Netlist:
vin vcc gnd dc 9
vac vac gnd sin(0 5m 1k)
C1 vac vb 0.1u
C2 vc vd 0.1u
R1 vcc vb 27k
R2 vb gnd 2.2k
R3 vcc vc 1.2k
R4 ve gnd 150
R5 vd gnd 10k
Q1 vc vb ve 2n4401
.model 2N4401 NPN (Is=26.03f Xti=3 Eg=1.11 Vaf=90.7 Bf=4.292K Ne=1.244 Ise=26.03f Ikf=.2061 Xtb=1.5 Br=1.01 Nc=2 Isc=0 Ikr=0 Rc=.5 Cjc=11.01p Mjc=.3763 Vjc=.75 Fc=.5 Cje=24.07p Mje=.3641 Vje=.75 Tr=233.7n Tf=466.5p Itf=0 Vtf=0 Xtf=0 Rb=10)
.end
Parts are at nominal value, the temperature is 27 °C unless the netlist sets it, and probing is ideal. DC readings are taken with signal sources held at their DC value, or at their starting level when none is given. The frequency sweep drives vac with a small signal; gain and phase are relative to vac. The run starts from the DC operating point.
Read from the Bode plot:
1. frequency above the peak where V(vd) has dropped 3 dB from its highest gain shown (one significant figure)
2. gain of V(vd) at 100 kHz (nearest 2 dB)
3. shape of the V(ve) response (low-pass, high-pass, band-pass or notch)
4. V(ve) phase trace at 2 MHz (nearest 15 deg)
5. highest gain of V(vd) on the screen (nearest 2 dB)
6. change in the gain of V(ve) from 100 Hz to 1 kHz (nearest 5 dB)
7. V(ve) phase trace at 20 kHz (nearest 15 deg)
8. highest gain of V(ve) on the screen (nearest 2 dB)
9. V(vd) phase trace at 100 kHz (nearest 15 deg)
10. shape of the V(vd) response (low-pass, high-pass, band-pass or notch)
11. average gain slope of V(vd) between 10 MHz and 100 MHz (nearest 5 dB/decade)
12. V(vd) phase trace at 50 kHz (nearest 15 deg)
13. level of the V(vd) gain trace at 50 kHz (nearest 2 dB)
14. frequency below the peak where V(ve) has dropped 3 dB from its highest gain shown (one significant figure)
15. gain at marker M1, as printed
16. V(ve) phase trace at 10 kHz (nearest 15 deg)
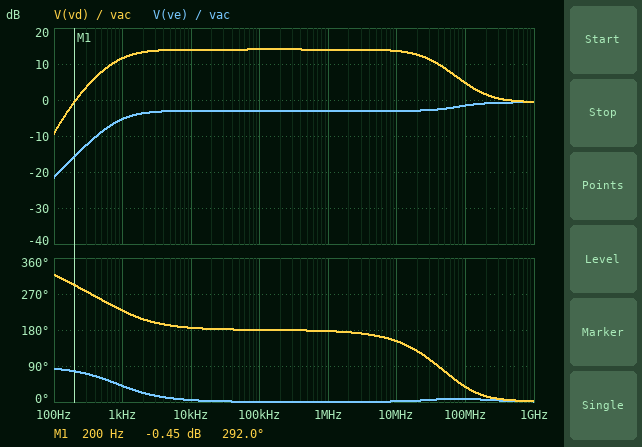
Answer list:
30 MHz
14 dB
high-pass
0 deg
14 dB
15 dB
0 deg
0 dB
180 deg
band-pass
-10 dB/decade
180 deg
14 dB
2 kHz
-0.45 dB
0 deg
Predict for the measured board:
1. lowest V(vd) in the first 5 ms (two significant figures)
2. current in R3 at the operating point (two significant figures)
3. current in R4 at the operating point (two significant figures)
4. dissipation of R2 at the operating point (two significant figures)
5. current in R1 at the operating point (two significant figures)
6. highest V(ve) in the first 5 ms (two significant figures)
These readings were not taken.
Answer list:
-19 mV
420 µA
430 µA
200 µW
310 µA
67 mV
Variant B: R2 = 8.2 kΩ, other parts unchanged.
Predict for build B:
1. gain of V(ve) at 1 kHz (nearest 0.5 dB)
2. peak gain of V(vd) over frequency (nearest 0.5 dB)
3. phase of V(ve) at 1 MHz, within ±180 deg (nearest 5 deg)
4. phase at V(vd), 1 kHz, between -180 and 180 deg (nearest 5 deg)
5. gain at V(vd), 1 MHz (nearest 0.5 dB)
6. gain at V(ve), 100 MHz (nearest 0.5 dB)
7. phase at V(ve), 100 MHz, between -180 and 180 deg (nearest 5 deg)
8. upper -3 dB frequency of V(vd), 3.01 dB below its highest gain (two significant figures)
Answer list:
-16.5 dB
8.5 dB
0 deg
-90 deg
6.5 dB
-1.0 dB
0 deg
1.4 MHz
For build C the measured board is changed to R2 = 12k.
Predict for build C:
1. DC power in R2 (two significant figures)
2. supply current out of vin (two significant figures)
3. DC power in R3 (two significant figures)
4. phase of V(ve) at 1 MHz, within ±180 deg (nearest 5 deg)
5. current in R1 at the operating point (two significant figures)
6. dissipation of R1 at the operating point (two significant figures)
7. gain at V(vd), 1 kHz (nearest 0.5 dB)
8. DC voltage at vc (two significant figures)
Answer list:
240 µW
6.8 mA
52 mW
0 deg
270 µA
2.0 mW
-23.0 dB
1.1 V
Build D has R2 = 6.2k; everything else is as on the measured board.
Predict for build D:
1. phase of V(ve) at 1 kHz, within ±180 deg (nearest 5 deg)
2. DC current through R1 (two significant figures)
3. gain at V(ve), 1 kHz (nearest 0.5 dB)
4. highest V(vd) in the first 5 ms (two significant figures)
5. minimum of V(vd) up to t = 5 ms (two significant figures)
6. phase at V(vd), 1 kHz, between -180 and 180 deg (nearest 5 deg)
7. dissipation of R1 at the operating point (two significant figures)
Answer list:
20 deg
280 µA
-1.0 dB
34 mV
-32 mV
-150 deg
2.1 mW
